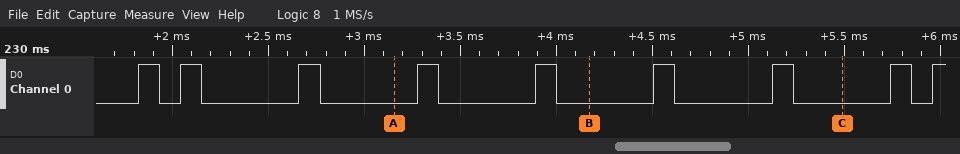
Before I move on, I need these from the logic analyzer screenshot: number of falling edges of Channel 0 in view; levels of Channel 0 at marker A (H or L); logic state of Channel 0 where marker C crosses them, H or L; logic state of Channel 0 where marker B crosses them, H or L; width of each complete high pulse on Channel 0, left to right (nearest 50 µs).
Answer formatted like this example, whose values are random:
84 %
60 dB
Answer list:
8
Channel 0=L
Channel 0=L
Channel 0=L
100 µs, 100 µs, 100 µs, 100 µs, 100 µs, 100 µs, 100 µs, 100 µs
